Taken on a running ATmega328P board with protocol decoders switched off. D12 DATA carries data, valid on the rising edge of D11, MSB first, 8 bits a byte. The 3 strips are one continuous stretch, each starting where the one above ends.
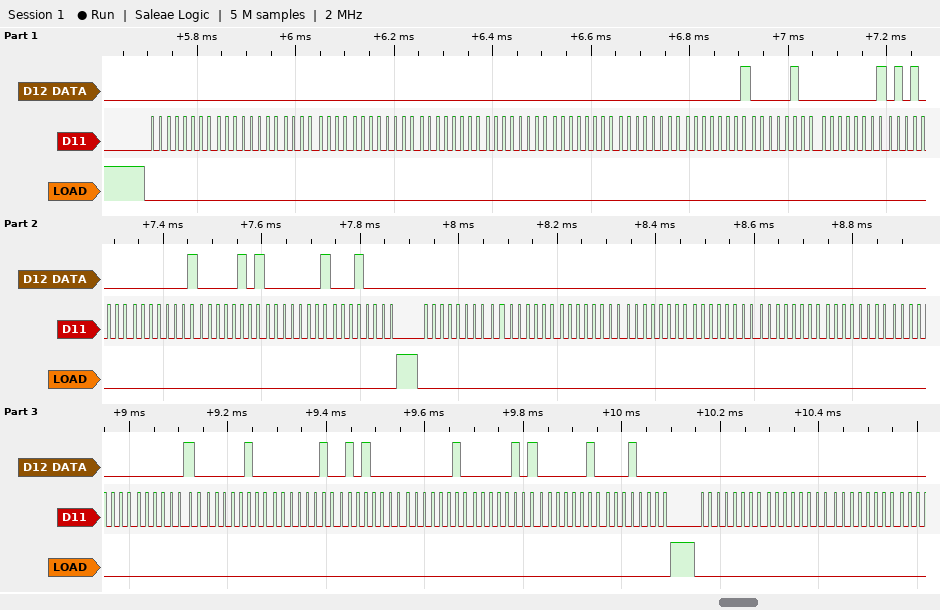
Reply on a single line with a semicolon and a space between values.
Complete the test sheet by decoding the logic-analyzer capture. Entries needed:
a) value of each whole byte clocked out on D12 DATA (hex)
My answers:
00 00 00 00 00 00 00 00 01 04 01 50 01 05 01 10 00 00 00 00 00 00 00 00 02 04 02 50 02 05 02 10 00 00 00
